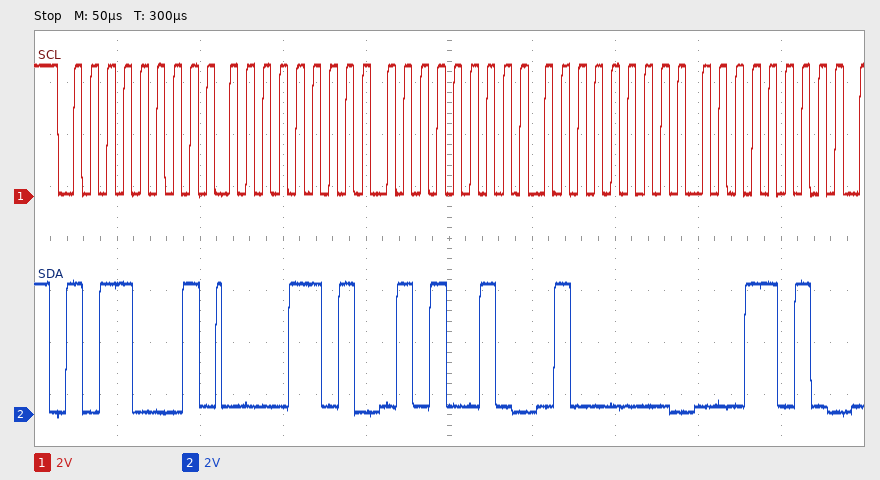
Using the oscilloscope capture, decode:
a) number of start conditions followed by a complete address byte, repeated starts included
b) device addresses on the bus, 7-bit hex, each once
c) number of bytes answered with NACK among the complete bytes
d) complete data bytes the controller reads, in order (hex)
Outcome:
1
0x58
0
0D 52 40 1A
